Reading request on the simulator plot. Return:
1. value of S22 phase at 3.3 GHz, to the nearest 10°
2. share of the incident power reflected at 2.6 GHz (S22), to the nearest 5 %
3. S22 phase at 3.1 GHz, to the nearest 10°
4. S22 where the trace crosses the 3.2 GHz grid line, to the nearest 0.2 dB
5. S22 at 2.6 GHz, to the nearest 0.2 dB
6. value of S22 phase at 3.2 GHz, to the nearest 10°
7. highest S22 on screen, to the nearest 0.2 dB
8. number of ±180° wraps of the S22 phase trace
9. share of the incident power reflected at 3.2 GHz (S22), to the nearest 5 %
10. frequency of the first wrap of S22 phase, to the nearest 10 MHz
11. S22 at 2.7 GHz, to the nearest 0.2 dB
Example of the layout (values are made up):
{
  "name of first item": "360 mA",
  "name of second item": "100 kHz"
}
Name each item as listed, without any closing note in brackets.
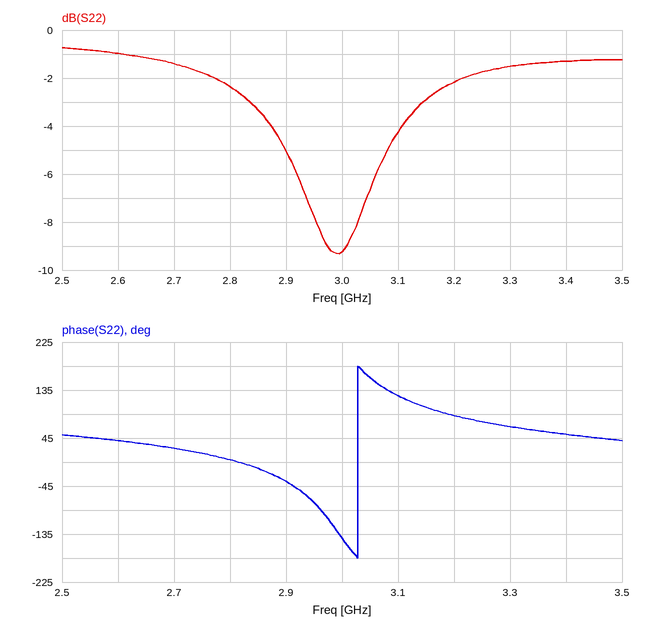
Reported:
{
  "value of S22 phase at 3.3 GHz, to the nearest 10°": "70°",
  "share of the incident power reflected at 2.6 GHz (S22), to the nearest 5 %": "80 %",
  "S22 phase at 3.1 GHz, to the nearest 10°": "120°",
  "S22 where the trace crosses the 3.2 GHz grid line, to the nearest 0.2 dB": "-2.2 dB",
  "S22 at 2.6 GHz, to the nearest 0.2 dB": "-1.0 dB",
  "value of S22 phase at 3.2 GHz, to the nearest 10°": "90°",
  "highest S22 on screen, to the nearest 0.2 dB": "-0.8 dB",
  "number of ±180° wraps of the S22 phase trace": "1",
  "share of the incident power reflected at 3.2 GHz (S22), to the nearest 5 %": "60 %",
  "frequency of the first wrap of S22 phase, to the nearest 10 MHz": "3.03 GHz",
  "S22 at 2.7 GHz, to the nearest 0.2 dB": "-1.4 dB"
}
